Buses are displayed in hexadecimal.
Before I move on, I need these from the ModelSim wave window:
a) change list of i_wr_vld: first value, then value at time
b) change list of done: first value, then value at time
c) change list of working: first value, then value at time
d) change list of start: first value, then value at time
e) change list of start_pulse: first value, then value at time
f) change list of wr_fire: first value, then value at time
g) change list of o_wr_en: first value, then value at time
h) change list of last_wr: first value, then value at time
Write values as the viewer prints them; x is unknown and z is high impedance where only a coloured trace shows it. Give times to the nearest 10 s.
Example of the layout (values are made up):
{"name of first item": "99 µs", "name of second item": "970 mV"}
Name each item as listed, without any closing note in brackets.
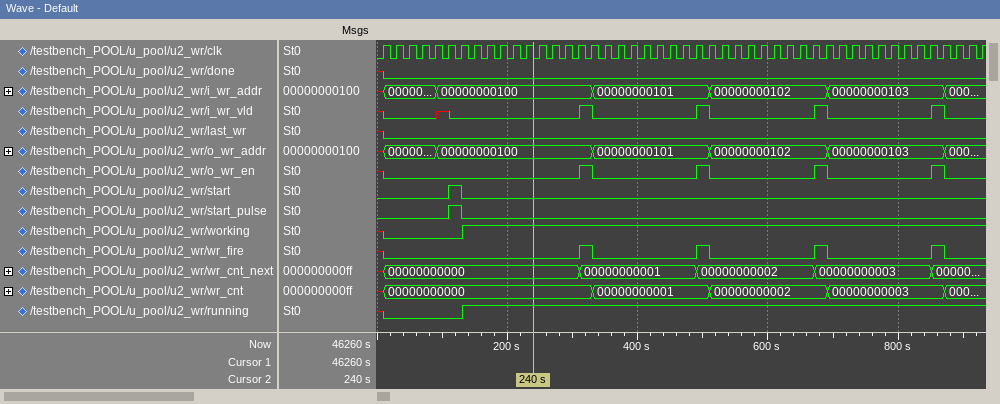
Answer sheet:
{"change list of i_wr_vld: first value, then value at time": "x, 0 at 10 s, x at 90 s, 0 at 110 s, 1 at 310 s, 0 at 330 s, 1 at 490 s, 0 at 510 s, 1 at 670 s, 0 at 690 s, 1 at 850 s, 0 at 870 s", "change list of done: first value, then value at time": "x, 0 at 10 s", "change list of working: first value, then value at time": "x, 0 at 10 s, 1 at 130 s", "change list of start: first value, then value at time": "0, 1 at 110 s, 0 at 130 s", "change list of start_pulse: first value, then value at time": "0, 1 at 110 s, 0 at 130 s", "change list of wr_fire: first value, then value at time": "x, 0 at 10 s, 1 at 310 s, 0 at 330 s, 1 at 490 s, 0 at 510 s, 1 at 670 s, 0 at 690 s, 1 at 850 s, 0 at 870 s", "change list of o_wr_en: first value, then value at time": "x, 0 at 10 s, 1 at 310 s, 0 at 330 s, 1 at 490 s, 0 at 510 s, 1 at 670 s, 0 at 690 s, 1 at 850 s, 0 at 870 s", "change list of last_wr: first value, then value at time": "x, 0 at 10 s"}
